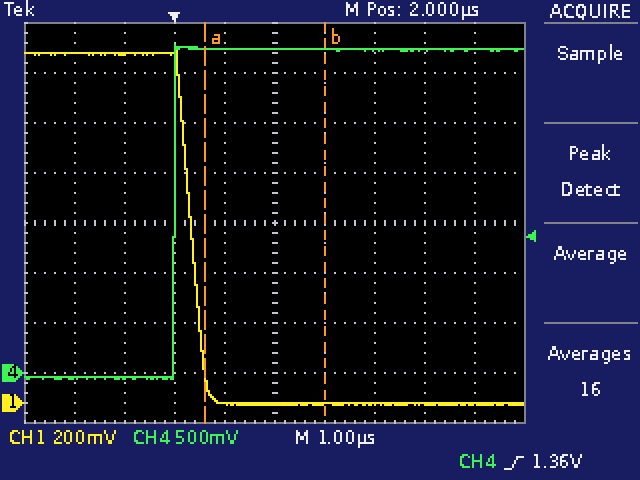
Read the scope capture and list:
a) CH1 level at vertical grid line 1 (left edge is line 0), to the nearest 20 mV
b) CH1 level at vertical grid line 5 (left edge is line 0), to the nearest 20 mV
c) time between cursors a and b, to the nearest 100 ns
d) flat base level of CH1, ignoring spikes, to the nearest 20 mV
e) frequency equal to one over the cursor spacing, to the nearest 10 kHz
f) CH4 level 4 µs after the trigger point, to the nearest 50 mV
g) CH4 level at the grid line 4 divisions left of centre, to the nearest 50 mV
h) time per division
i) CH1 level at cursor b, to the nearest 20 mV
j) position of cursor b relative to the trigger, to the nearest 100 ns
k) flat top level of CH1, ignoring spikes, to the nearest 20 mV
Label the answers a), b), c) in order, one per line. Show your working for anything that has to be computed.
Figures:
a) 1.40 V
b) 0 mV
c) 2.4 µs
d) 0 mV
e) 1 / 2.4 µs ≈ 420 kHz
f) 3.25 V
g) -50 mV
h) 1 µs
i) 0 mV
j) +3.0 µs
k) 1.40 V
